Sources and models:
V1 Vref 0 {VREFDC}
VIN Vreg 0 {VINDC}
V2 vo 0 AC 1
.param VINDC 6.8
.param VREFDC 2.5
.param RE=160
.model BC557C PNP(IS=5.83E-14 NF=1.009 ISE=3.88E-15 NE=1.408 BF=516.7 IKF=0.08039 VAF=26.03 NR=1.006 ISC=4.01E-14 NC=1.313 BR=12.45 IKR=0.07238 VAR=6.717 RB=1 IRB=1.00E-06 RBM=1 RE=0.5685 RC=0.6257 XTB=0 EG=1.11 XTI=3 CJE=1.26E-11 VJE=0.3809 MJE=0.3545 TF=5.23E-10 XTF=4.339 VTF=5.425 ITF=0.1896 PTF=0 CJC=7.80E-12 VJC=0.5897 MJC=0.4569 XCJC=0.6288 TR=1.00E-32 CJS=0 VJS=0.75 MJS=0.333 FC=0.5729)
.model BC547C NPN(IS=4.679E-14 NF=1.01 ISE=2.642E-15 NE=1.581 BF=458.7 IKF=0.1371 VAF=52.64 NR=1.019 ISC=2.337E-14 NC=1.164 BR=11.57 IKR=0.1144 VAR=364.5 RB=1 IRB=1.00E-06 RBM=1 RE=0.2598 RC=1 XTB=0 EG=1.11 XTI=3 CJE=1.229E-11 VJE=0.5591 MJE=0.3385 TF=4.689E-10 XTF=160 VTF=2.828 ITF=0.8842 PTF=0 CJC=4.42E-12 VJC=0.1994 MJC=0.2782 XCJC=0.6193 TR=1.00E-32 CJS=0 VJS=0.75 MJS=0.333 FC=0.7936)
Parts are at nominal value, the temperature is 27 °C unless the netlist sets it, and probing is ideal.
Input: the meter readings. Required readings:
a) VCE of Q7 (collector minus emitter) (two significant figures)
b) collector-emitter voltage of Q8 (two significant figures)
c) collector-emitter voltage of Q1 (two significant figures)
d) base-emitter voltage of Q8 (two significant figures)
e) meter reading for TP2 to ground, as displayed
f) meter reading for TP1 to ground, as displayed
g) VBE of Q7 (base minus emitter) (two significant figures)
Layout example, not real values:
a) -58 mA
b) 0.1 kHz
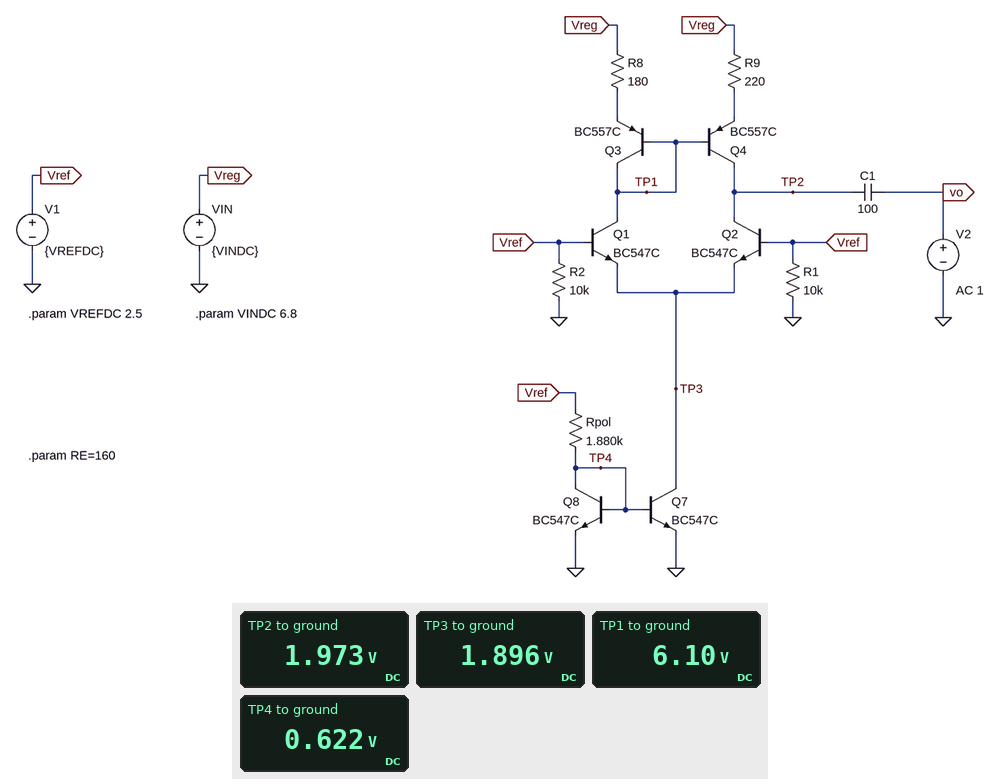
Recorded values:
a) 1.9 V
b) 620 mV
c) 4.2 V
d) 620 mV
e) 1.973 V
f) 6.10 V
g) 620 mV
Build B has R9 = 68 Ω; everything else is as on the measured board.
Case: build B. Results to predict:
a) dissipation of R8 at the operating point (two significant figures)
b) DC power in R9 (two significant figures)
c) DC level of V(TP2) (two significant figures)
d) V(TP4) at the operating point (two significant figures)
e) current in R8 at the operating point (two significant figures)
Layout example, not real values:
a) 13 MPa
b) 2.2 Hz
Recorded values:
a) 31 µW
b) 24 µW
c) 6.7 V
d) 620 mV
e) 420 µA
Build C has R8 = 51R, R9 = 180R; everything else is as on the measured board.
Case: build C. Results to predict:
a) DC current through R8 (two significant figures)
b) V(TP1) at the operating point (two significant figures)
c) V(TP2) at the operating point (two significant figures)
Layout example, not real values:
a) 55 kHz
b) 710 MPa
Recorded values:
a) 660 µA
b) 6.2 V
c) 1.9 V
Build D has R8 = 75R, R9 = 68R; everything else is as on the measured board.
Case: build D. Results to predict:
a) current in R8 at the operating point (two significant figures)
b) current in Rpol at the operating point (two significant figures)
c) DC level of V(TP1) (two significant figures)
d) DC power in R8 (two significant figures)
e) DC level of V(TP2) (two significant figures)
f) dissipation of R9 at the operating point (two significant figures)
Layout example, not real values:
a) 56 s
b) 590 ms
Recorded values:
a) 500 µA
b) 1.0 mA
c) 6.2 V
d) 19 µW
e) 6.7 V
f) 18 µW
